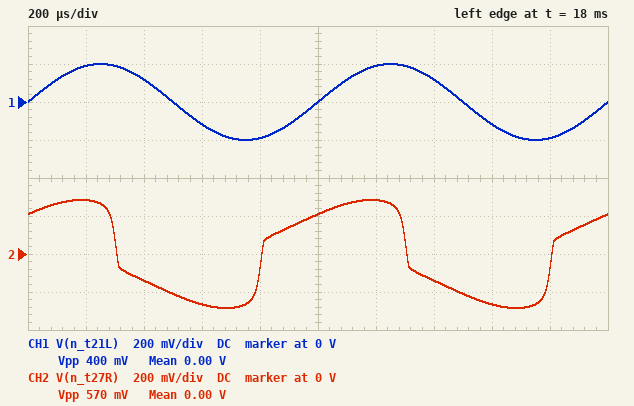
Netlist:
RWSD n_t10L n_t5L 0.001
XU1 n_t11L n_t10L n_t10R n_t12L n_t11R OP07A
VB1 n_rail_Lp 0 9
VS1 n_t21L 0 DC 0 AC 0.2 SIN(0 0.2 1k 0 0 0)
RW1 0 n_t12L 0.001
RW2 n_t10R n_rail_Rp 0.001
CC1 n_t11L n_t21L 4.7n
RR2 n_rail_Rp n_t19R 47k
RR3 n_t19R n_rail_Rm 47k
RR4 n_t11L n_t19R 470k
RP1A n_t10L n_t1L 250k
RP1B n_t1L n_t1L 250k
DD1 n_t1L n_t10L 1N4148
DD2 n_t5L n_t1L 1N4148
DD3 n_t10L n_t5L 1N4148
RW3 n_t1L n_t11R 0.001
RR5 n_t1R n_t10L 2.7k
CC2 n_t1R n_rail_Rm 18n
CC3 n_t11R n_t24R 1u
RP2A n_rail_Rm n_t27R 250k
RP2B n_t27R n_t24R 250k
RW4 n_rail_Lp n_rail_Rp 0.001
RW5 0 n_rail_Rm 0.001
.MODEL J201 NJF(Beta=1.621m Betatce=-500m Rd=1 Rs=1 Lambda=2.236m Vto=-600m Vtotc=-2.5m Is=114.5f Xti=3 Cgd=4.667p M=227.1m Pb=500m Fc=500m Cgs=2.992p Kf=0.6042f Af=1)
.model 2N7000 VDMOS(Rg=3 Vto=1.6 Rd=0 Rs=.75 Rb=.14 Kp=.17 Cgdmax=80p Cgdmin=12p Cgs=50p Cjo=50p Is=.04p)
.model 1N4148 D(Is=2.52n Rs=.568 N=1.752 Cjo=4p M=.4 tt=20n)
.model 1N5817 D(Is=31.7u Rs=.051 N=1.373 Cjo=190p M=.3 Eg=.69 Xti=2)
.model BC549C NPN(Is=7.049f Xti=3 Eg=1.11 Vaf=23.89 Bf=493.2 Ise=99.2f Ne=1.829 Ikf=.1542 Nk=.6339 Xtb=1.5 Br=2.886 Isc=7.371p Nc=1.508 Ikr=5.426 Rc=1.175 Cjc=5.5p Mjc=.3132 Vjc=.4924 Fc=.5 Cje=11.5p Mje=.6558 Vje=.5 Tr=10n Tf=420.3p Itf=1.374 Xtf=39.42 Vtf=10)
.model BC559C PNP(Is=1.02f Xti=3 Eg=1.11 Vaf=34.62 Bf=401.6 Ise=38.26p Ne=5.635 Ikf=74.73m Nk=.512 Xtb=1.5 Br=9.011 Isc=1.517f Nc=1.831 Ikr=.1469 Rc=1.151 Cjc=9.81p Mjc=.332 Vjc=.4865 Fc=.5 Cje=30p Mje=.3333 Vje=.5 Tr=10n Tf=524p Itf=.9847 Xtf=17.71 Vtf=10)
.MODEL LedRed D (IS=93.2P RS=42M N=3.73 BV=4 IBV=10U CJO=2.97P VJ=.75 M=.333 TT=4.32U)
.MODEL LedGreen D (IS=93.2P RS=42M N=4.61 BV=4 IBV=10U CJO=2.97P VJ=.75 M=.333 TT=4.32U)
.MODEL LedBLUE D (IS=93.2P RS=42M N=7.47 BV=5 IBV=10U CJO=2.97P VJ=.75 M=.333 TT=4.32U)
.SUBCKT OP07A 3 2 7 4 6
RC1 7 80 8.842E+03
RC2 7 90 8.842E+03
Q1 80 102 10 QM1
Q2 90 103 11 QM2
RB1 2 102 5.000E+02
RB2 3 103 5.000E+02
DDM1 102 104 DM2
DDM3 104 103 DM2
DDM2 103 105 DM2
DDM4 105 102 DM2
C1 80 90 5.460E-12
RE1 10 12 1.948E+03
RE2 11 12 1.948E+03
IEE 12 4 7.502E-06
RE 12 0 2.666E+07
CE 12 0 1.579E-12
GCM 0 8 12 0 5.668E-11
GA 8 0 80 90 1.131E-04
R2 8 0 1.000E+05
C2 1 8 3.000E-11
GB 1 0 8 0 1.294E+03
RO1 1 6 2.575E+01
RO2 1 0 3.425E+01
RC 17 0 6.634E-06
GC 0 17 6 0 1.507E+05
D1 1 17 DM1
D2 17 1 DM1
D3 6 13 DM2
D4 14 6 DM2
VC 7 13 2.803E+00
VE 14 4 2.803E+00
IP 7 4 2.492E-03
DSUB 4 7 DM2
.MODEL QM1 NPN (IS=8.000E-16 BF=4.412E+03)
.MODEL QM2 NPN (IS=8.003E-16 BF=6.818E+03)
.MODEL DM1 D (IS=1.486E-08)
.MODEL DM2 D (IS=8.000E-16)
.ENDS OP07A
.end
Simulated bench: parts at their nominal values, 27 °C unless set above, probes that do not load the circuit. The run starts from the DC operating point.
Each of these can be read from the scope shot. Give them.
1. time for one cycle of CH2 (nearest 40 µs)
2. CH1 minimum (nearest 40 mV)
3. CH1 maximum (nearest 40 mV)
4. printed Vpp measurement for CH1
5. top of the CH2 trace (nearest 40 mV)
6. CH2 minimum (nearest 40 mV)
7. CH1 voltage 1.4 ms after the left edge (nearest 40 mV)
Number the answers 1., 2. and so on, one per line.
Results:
1. 1.00 ms
2. -200 mV
3. 200 mV
4. 400 mV
5. 280 mV
6. -280 mV
7. 120 mV
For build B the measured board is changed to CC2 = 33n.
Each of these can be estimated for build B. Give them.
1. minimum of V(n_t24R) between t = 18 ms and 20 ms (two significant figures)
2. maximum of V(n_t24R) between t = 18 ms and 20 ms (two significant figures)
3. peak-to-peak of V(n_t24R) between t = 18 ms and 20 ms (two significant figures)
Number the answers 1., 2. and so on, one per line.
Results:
1. -610 mV
2. 610 mV
3. 1.2 V
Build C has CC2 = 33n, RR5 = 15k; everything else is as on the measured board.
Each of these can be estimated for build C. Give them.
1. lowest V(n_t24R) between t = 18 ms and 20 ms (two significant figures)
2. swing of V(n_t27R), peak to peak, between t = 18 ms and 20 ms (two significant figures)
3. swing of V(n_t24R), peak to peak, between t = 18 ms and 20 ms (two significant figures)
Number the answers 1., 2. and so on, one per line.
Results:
1. -580 mV
2. 580 mV
3. 1.2 V
